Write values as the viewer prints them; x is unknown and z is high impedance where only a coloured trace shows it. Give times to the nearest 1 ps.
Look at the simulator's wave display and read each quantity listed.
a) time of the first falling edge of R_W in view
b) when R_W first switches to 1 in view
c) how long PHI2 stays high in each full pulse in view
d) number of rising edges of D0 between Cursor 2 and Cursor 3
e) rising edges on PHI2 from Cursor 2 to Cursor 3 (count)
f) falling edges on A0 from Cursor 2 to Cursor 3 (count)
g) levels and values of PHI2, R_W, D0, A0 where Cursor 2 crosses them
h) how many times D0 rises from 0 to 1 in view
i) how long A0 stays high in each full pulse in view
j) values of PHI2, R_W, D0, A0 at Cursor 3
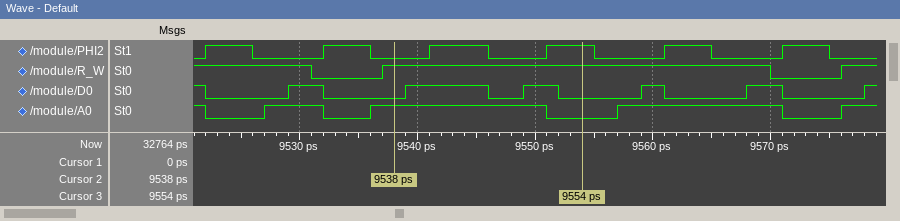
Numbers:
9531 ps
9537 ps
4 ps, 4 ps, 5 ps, 4 ps, 4 ps, 4 ps
2
2
1
PHI2=0, R_W=1, D0=0, A0=1
6
5 ps, 15 ps, 14 ps
PHI2=1, R_W=1, D0=0, A0=0
